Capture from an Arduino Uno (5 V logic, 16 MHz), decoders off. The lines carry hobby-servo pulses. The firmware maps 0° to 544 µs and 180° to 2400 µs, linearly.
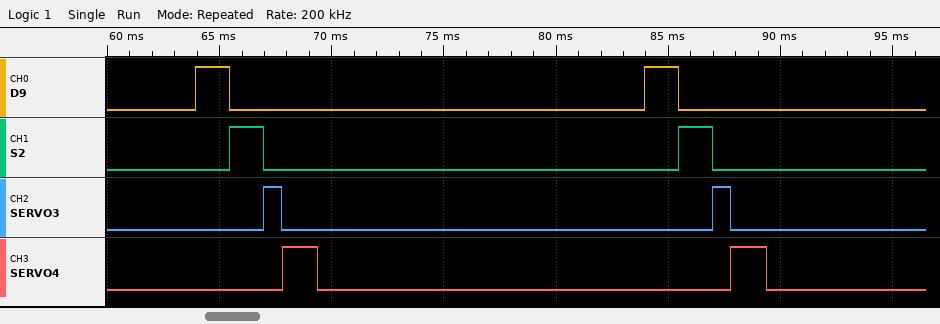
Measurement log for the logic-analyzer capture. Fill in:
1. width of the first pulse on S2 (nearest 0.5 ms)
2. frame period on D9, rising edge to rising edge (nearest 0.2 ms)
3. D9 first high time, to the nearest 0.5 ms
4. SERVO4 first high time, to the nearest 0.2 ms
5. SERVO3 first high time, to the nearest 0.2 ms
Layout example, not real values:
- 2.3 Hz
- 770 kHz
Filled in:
- 1.5 ms
- 20.0 ms
- 1.5 ms
- 1.6 ms
- 0.8 ms
